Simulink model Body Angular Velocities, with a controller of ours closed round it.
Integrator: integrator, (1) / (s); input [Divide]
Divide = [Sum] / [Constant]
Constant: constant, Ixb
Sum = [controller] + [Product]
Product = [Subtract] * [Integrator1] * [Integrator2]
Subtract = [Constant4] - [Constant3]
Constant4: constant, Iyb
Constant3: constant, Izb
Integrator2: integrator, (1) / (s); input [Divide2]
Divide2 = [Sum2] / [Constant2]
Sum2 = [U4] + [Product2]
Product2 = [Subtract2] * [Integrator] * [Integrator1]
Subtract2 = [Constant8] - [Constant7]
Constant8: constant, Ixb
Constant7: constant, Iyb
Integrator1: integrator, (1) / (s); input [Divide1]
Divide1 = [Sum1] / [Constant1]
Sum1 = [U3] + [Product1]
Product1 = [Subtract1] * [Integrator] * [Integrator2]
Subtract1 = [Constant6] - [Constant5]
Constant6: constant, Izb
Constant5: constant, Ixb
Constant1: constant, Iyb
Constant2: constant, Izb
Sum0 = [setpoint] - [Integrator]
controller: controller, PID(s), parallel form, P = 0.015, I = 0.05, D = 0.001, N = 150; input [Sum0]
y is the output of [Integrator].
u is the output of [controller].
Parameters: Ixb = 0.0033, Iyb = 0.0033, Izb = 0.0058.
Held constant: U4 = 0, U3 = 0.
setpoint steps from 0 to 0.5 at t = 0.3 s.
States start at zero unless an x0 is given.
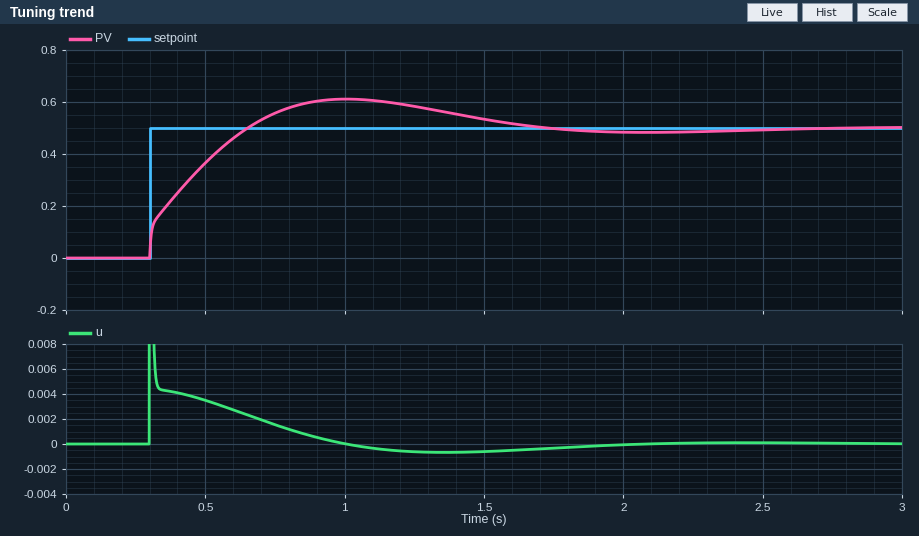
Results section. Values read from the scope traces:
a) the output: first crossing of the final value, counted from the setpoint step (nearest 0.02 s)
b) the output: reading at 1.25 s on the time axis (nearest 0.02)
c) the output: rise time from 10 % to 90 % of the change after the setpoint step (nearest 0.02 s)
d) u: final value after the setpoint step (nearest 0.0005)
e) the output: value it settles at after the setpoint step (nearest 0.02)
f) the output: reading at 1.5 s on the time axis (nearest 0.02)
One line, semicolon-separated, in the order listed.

0.36 s; 0.58; 0.28 s; 0.0000; 0.50; 0.54
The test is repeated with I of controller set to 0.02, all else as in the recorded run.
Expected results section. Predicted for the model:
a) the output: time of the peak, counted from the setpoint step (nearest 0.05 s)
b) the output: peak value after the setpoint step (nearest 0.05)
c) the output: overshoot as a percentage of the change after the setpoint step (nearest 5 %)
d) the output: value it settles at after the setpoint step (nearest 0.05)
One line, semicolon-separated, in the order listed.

1.00 s; 0.55; 15 %; 0.50
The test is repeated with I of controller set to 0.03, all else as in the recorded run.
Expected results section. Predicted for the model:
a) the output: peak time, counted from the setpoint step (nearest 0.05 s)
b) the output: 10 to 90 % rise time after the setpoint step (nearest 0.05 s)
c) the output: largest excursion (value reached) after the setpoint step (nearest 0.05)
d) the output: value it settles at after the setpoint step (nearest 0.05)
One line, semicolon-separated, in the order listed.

0.85 s; 0.35 s; 0.60; 0.50
